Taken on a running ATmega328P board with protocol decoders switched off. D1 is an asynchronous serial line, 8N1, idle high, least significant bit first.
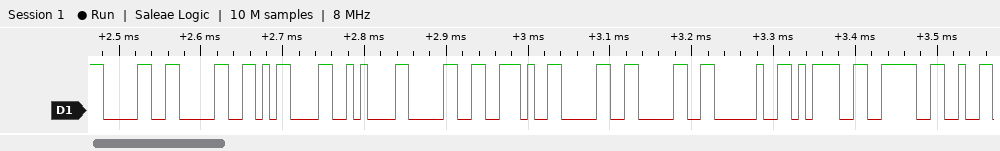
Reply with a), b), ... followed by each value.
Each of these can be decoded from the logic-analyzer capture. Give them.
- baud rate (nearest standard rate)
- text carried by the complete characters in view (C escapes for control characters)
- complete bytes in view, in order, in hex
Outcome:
a) 115200 baud
b) "00\r\n0.00 =>"
c) 30 30 0D 0A 30 2E 30 30 20 3D 3E
